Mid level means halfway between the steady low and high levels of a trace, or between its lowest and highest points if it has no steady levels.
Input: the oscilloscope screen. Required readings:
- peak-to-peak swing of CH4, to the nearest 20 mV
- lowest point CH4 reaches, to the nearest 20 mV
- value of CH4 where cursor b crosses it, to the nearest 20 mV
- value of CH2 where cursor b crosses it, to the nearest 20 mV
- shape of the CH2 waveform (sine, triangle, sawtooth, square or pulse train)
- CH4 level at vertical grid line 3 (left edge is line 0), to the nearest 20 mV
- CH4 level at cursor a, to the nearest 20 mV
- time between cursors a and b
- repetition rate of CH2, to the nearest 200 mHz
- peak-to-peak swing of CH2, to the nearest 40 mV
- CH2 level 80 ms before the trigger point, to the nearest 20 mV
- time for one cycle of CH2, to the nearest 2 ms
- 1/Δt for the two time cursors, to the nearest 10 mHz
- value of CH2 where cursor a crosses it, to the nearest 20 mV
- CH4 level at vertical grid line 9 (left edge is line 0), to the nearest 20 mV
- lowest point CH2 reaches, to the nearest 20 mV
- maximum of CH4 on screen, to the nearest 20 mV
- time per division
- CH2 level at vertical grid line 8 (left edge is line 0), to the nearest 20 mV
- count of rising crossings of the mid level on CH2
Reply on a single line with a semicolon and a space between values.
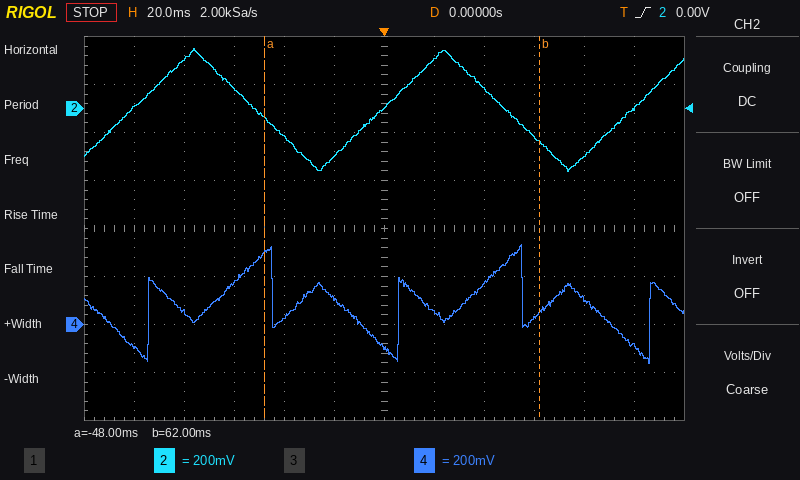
500 mV; -160 mV; 60 mV; -140 mV; triangle; 180 mV; 300 mV; 110 ms; 10.0 Hz; 520 mV; 200 mV; 100 ms; 9.09 Hz; -40 mV; 20 mV; -260 mV; 340 mV; 20 ms; 80 mV; 3
